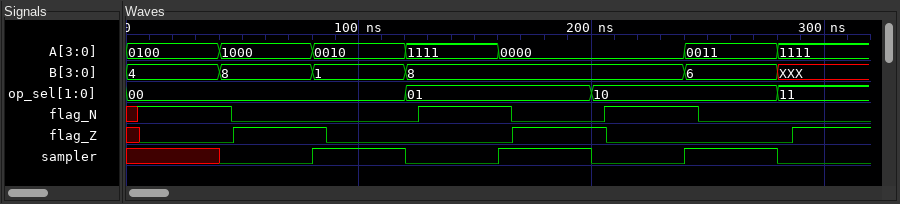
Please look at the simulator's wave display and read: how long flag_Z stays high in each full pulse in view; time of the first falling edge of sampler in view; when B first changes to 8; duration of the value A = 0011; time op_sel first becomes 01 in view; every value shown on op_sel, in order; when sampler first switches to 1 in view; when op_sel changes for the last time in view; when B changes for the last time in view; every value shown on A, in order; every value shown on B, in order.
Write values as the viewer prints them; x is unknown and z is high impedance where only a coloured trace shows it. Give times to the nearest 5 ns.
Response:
40 ns, 40 ns
120 ns
40 ns
40 ns
120 ns
00, 01, 10, 11
80 ns
280 ns
280 ns
0100, 1000, 0010, 1111, 0000, 0011, 1111
4, 8, 1, 8, 6, XXX
